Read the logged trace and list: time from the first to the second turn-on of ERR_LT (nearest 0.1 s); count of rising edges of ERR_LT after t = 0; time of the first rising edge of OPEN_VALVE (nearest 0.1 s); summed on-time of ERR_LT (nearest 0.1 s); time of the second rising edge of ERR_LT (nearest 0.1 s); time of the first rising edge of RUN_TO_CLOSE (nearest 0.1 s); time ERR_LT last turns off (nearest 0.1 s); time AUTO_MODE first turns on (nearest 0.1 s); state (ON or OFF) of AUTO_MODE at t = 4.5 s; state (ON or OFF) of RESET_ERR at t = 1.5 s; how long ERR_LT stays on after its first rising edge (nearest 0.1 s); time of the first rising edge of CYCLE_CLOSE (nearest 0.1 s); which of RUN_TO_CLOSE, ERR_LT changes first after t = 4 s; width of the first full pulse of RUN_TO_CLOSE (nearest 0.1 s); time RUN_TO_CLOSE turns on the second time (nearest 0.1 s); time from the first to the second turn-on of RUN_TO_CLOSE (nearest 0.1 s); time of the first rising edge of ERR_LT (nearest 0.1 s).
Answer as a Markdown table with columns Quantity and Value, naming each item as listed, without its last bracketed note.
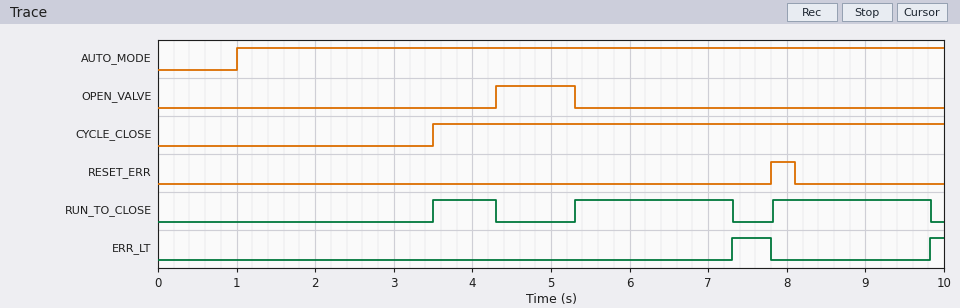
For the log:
| Quantity | Value |
|---|---|
| time from the first to the second turn-on of ERR_LT | 2.5 s |
| count of rising edges of ERR_LT after t = 0 | 2 |
| time of the first rising edge of OPEN_VALVE | 4.3 s |
| summed on-time of ERR_LT | 0.7 s |
| time of the second rising edge of ERR_LT | 9.8 s |
| time of the first rising edge of RUN_TO_CLOSE | 3.5 s |
| time ERR_LT last turns off | 7.8 s |
| time AUTO_MODE first turns on | 1.0 s |
| state (ON or OFF) of AUTO_MODE at t = 4.5 s | ON |
| state (ON or OFF) of RESET_ERR at t = 1.5 s | OFF |
| how long ERR_LT stays on after its first rising edge | 0.5 s |
| time of the first rising edge of CYCLE_CLOSE | 3.5 s |
| which of RUN_TO_CLOSE, ERR_LT changes first after t = 4 s | RUN_TO_CLOSE |
| width of the first full pulse of RUN_TO_CLOSE | 0.8 s |
| time RUN_TO_CLOSE turns on the second time | 5.3 s |
| time from the first to the second turn-on of RUN_TO_CLOSE | 1.8 s |
| time of the first rising edge of ERR_LT | 7.3 s |
